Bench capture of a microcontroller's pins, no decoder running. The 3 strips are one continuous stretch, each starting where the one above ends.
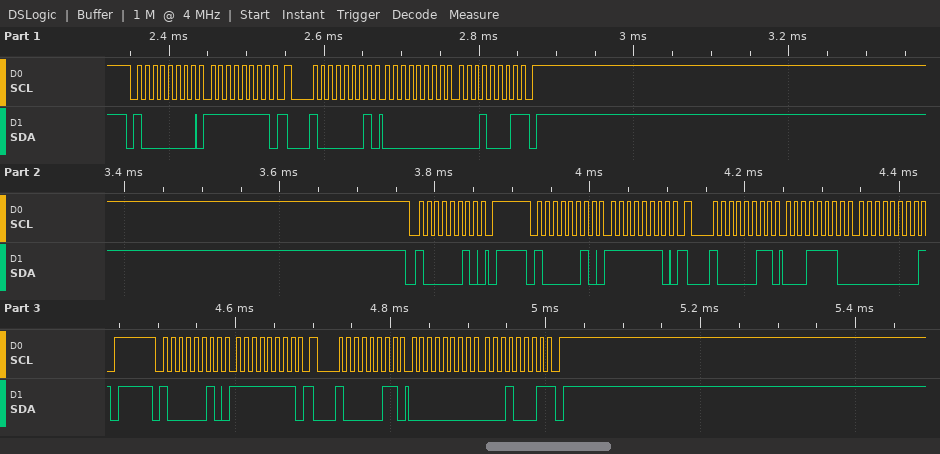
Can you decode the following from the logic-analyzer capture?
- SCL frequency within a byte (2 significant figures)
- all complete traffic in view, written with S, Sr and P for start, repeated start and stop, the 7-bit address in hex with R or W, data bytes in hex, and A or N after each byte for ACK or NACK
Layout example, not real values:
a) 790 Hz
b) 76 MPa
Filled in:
a) 100 kHz
b) S 40W A FF A Sr 40R A 00 A 11 N P S 41W A P S 41W A FE A Sr 41R A 1E A 00 N P S 41W A FF A Sr 41R A 00 A 11 N P
